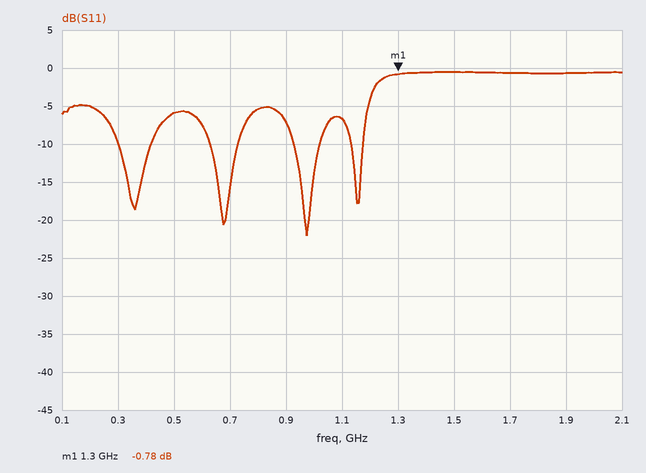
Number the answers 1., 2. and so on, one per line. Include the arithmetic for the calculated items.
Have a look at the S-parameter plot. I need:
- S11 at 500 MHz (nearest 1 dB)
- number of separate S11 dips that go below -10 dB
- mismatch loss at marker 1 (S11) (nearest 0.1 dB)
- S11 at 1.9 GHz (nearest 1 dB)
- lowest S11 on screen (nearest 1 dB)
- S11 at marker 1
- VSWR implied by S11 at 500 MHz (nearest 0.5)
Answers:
1. -6 dB
2. 4
3. −10 log10(1 − 10^(-0.78/10)) ≈ 7.8 dB
4. -1 dB
5. -22 dB
6. -0.78 dB
7. |Γ| = 10^(-6/20) = 0.5012; VSWR = (1 + 0.5012)/(1 − 0.5012) ≈ 3.0
